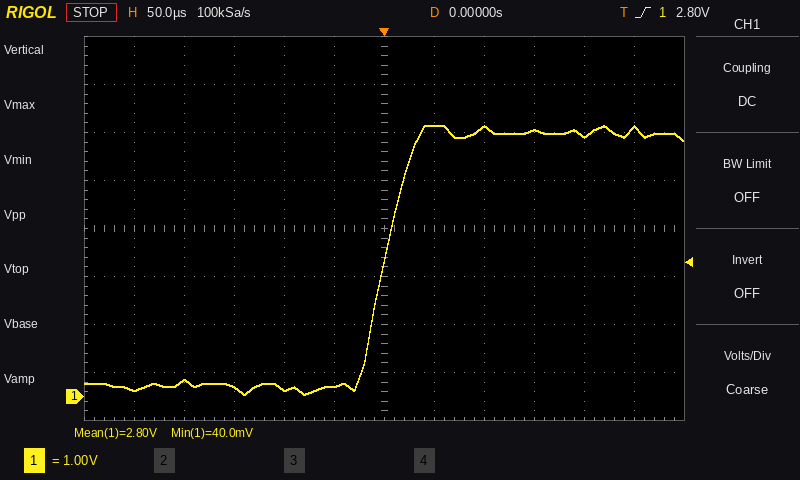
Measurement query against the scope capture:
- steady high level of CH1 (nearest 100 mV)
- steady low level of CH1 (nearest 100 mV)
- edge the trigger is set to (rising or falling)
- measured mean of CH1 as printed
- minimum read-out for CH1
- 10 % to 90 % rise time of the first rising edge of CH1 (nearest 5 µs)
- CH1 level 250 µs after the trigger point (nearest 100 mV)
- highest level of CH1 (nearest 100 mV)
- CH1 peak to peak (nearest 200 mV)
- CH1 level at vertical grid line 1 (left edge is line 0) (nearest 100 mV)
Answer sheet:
5.5 V
200 mV
rising
2.80 V
40.0 mV
45 µs
5.6 V
5.6 V
5.6 V
100 mV
